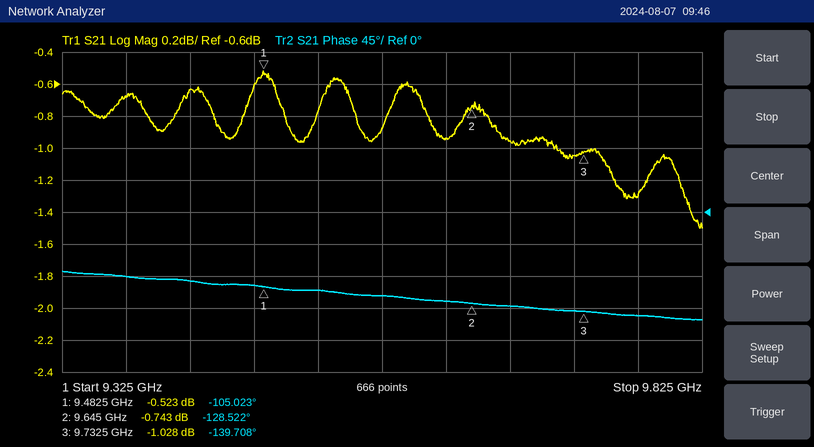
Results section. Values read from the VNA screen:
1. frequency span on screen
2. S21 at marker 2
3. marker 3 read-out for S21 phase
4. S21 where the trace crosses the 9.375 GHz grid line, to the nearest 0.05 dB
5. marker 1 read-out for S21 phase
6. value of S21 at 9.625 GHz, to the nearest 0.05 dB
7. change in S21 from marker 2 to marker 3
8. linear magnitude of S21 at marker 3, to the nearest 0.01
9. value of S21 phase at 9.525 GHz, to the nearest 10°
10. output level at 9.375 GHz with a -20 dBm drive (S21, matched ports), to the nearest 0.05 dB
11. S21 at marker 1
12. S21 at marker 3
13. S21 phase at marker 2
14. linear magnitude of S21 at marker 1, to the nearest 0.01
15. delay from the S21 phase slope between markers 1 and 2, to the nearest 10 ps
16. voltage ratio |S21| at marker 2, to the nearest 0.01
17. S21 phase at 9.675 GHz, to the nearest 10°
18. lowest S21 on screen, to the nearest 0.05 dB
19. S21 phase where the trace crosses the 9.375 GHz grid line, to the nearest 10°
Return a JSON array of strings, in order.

["500 MHz", "-0.743 dB", "-139.708°", "-0.70 dB", "-105.023°", "-0.95 dB", "-0.285 dB", "0.89", "-110°", "-20.70 dBm", "-0.523 dB", "-1.028 dB", "-128.522°", "0.94", "400 ps", "0.92", "-130°", "-1.50 dB", "-90°"]
